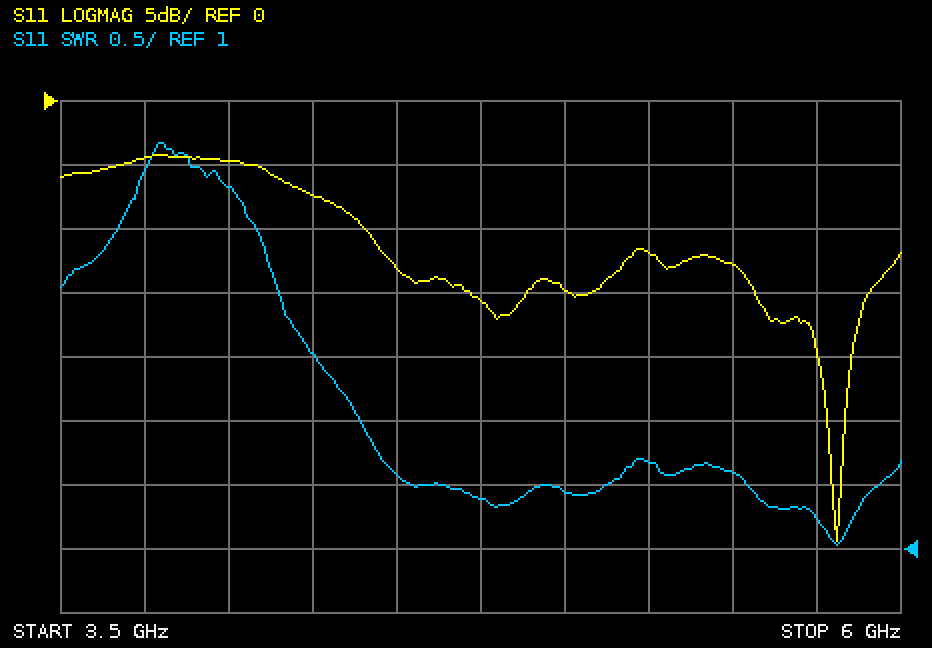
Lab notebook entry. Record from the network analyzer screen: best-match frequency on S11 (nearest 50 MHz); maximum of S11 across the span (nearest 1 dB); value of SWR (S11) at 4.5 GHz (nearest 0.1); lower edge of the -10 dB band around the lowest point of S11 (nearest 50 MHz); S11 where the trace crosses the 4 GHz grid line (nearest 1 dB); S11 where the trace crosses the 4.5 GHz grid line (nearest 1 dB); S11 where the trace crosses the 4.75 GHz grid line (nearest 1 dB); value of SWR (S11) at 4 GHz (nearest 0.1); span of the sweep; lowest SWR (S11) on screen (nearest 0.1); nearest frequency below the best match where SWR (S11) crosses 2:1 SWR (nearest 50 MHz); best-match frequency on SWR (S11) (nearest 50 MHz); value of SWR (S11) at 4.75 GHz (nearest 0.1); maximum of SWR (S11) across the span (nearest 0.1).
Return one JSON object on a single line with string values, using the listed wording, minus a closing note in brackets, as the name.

{"best-match frequency on S11": "5.80 GHz", "maximum of S11 across the span": "-4 dB", "value of SWR (S11) at 4.5 GHz": "1.6", "lower edge of the -10 dB band around the lowest point of S11": "4.40 GHz", "S11 where the trace crosses the 4 GHz grid line": "-5 dB", "S11 where the trace crosses the 4.5 GHz grid line": "-13 dB", "S11 where the trace crosses the 4.75 GHz grid line": "-16 dB", "value of SWR (S11) at 4 GHz": "3.8", "span of the sweep": "2.5 GHz", "lowest SWR (S11) on screen": "1.0", "nearest frequency below the best match where SWR (S11) crosses 2:1 SWR": "4.40 GHz", "best-match frequency on SWR (S11)": "5.80 GHz", "value of SWR (S11) at 4.75 GHz": "1.4", "maximum of SWR (S11) across the span": "4.2"}
